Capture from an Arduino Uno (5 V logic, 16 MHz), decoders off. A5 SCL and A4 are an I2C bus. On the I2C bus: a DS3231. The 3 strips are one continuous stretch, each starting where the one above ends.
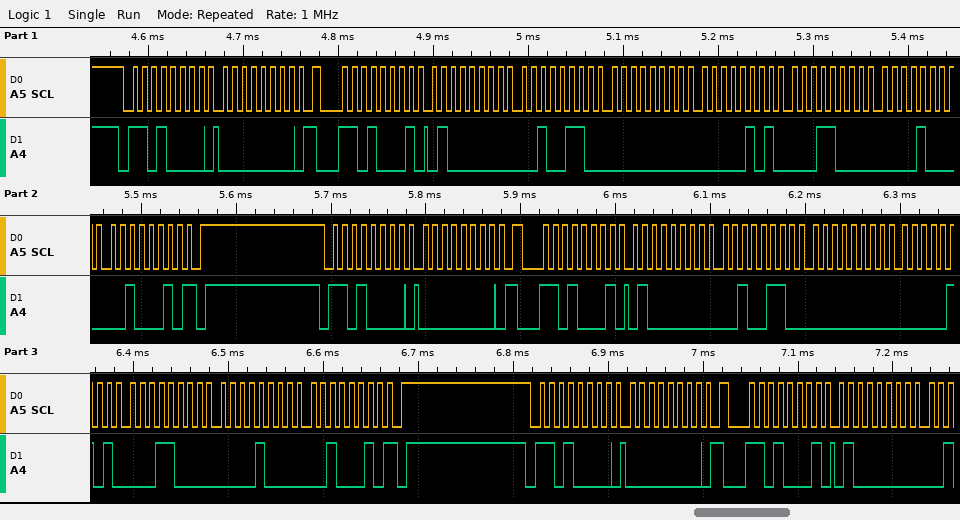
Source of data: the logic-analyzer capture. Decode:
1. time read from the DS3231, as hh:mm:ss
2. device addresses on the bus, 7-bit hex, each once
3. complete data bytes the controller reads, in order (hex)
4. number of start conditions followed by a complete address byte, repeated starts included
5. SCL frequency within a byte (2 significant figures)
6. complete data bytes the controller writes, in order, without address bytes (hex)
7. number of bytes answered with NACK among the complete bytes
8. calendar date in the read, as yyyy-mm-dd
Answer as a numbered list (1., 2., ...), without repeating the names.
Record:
1. 00:26:40
2. 0x68
3. 40 26 00 05 18 08 22 40 26 00 05 18 08 22 40
4. 6
5. 100 kHz
6. 00 00 00
7. 2
8. 2022-08-18
